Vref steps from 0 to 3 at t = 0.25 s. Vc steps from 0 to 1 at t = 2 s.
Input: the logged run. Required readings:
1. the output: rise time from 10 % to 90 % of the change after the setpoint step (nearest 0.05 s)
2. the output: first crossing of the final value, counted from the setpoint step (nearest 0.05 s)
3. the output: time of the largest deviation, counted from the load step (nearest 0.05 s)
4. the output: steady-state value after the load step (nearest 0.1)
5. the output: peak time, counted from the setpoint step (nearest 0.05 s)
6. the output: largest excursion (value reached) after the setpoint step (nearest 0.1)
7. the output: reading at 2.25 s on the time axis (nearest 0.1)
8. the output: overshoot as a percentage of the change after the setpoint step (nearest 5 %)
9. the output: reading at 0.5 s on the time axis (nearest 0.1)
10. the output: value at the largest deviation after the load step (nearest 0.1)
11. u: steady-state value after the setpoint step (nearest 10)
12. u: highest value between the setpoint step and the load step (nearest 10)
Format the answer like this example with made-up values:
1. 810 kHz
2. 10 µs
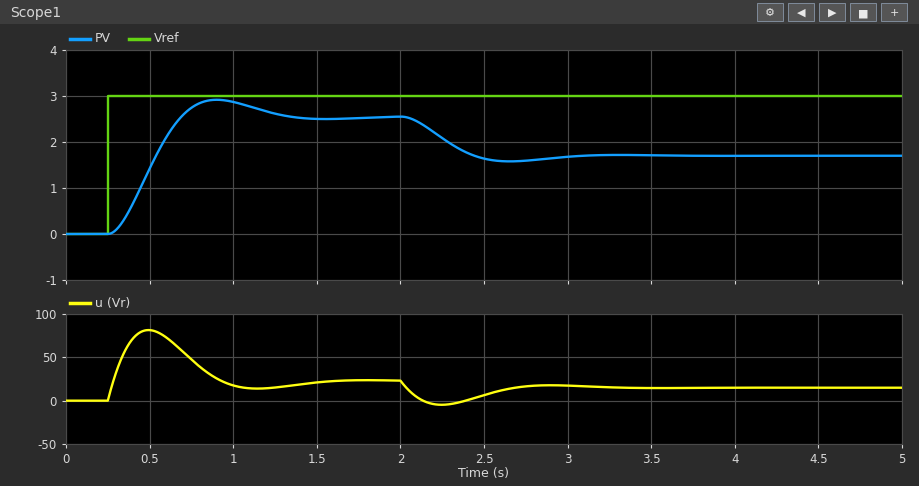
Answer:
1. 0.30 s
2. 0.45 s
3. 0.65 s
4. 1.7
5. 0.65 s
6. 2.9
7. 2.1
8. 15 %
9. 1.4
10. 1.6
11. 20
12. 80
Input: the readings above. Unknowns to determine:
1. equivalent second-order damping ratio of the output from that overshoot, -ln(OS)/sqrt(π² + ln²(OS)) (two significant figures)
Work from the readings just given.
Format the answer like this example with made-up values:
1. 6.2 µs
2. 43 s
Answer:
1. 0.52
